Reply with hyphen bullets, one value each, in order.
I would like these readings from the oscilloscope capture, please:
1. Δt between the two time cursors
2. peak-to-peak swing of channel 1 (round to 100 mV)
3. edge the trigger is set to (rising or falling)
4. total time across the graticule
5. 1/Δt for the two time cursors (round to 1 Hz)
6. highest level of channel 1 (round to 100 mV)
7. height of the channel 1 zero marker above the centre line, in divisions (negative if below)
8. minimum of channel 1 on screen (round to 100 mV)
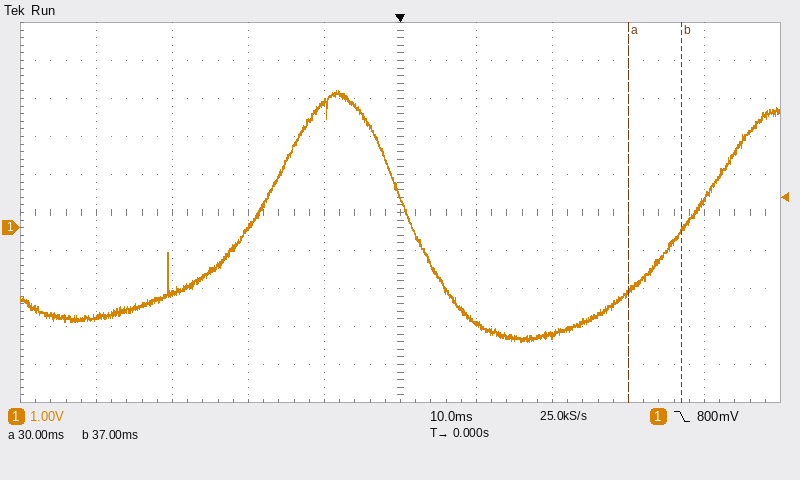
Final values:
- 7 ms
- 6.6 V
- falling
- 100 ms
- 143 Hz
- 3.6 V
- -0.4 div
- -3.0 V
